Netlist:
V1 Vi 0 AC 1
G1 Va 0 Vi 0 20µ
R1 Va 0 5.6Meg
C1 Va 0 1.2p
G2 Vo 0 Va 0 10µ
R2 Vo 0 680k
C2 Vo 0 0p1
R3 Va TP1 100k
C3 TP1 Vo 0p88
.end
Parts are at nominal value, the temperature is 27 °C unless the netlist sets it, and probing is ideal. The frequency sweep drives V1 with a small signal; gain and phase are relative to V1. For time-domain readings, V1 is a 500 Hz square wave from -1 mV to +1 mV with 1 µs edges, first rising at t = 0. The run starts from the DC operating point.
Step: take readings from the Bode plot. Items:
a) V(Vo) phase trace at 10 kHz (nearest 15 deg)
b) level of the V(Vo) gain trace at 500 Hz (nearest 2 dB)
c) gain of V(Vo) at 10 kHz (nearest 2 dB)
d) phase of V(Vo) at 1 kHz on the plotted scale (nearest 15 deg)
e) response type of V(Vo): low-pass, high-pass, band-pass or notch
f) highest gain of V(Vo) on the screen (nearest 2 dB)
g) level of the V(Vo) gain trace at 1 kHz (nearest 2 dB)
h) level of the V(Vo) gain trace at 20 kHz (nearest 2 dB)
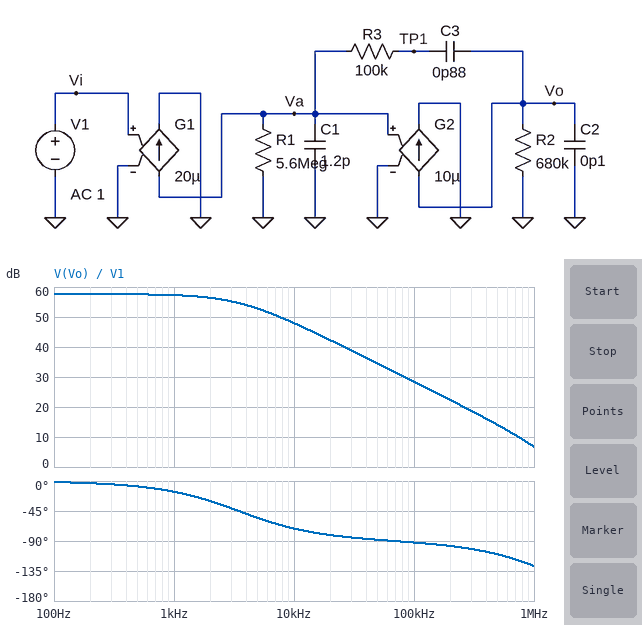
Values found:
-75 deg
58 dB
48 dB
-15 deg
low-pass
58 dB
58 dB
42 dB
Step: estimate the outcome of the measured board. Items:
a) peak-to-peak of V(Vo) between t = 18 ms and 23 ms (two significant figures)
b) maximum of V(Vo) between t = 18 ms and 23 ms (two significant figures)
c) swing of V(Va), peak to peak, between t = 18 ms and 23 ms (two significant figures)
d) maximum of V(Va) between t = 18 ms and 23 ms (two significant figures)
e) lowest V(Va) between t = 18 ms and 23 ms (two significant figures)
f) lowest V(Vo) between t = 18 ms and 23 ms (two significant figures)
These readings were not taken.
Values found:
1.5 V
760 mV
220 mV
110 mV
-110 mV
-760 mV
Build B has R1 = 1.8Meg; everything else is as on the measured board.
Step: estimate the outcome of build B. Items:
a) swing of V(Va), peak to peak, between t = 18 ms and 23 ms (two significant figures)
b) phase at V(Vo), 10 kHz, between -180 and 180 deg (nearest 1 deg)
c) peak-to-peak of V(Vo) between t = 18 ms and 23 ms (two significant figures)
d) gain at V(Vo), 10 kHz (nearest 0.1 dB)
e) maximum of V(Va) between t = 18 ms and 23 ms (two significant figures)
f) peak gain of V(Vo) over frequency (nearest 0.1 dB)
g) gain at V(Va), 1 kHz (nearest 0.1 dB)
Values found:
72 mV
-44 deg
490 mV
45.0 dB
36 mV
47.8 dB
31.1 dB
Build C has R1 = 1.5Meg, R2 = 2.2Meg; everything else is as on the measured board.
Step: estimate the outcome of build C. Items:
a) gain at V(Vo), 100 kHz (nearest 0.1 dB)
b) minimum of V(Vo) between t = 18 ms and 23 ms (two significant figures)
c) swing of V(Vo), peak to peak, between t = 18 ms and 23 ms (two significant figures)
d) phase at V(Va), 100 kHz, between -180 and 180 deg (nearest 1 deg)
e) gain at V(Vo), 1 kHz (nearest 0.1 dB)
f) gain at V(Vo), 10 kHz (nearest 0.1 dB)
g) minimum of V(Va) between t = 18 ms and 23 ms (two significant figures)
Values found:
29.7 dB
-660 mV
1.3 V
143 deg
56.2 dB
48.9 dB
-30 mV
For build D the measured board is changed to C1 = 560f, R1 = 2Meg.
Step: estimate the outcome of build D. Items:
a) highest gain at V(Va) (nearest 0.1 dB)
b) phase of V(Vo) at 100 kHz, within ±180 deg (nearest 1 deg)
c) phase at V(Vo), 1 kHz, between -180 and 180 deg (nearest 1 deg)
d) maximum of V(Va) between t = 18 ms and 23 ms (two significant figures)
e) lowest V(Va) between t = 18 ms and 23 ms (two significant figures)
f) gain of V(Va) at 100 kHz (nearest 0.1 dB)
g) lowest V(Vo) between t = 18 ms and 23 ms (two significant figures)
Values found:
32.0 dB
-86 deg
-6 deg
40 mV
-40 mV
13.1 dB
-270 mV
